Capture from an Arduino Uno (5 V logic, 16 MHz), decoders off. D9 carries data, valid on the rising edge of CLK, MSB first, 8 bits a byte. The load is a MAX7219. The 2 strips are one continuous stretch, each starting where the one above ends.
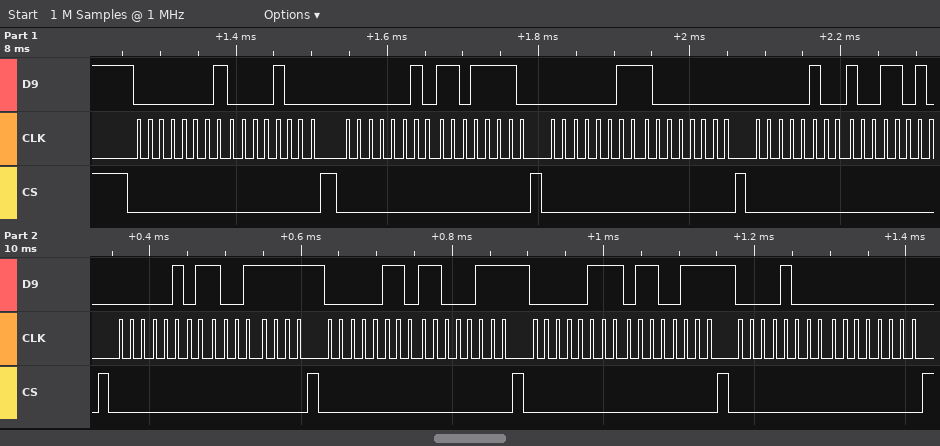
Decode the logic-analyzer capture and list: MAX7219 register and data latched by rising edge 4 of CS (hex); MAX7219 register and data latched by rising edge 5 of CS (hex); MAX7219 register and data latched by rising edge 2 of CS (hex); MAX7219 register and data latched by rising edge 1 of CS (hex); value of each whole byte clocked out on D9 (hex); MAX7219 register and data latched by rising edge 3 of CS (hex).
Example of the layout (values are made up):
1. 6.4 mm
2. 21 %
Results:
1. register 0x4, data 0x9A
2. register 0x5, data 0x9F
3. register 0x2, data 0xDE
4. register 0x1, data 0x08
5. 01 08 02 DE 03 80 04 9A 05 9F 06 C7 07 67 08 00
6. register 0x3, data 0x80
